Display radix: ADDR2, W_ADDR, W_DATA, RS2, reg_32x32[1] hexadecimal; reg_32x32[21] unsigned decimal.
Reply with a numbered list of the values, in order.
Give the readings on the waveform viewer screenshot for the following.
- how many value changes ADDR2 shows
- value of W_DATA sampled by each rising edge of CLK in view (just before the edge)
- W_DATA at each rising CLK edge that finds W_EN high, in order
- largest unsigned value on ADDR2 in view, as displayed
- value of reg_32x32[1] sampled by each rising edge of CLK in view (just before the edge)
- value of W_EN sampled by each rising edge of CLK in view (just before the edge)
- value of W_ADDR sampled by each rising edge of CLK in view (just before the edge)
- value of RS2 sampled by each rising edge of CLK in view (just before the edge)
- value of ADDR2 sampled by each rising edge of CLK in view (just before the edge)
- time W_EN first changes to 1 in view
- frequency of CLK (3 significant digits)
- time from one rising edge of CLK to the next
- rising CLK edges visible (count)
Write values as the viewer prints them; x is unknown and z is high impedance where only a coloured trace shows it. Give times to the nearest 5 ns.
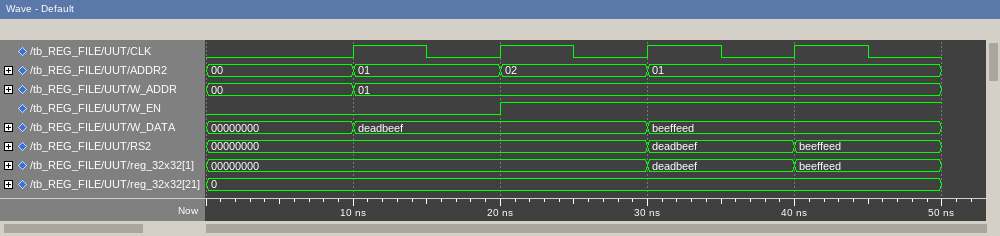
1. 3
2. 00000000, deadbeef, deadbeef, beeffeed
3. deadbeef, beeffeed
4. 02
5. 00000000, 00000000, 00000000, deadbeef
6. 0 0 1 1
7. 00, 01, 01, 01
8. 00000000, 00000000, 00000000, deadbeef
9. 00, 01, 02, 01
10. 20 ns
11. 100 MHz
12. 10 ns
13. 4
